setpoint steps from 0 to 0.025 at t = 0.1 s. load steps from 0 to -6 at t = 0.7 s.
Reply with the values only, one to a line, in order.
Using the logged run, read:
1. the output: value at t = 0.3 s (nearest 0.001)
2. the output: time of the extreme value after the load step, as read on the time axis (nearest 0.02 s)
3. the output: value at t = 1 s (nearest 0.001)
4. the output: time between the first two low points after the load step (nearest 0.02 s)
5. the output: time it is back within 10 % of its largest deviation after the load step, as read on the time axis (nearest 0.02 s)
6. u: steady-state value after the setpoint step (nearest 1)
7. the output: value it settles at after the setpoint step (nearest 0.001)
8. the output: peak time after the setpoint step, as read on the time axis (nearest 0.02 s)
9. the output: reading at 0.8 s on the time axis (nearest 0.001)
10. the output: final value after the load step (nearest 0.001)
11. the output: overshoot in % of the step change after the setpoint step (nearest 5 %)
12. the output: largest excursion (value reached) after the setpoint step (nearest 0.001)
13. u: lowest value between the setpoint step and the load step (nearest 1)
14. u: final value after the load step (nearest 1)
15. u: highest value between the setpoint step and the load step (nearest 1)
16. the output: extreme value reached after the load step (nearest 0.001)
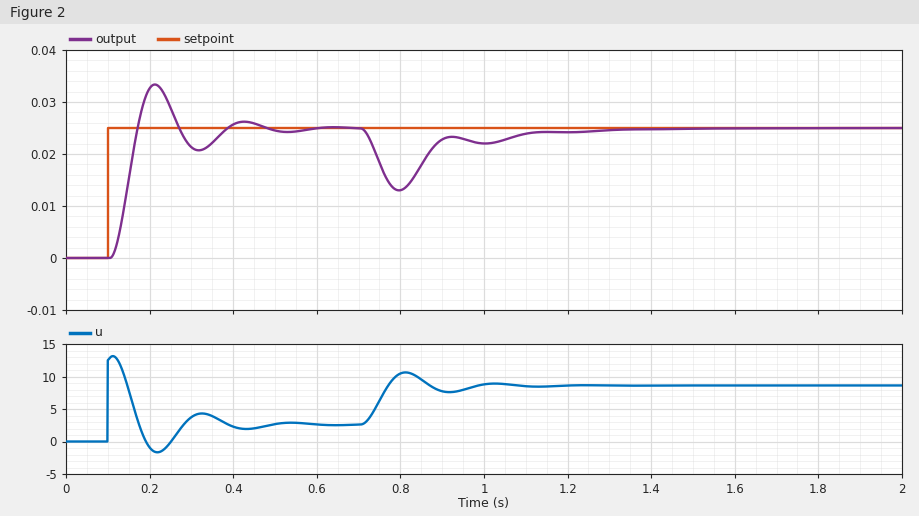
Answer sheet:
0.021
0.80 s
0.022
0.20 s
1.10 s
3
0.025
0.22 s
0.013
0.025
35 %
0.033
-2
9
13
0.013
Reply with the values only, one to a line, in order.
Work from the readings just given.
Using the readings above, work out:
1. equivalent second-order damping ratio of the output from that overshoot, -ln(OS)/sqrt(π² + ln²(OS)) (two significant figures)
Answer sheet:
0.32
